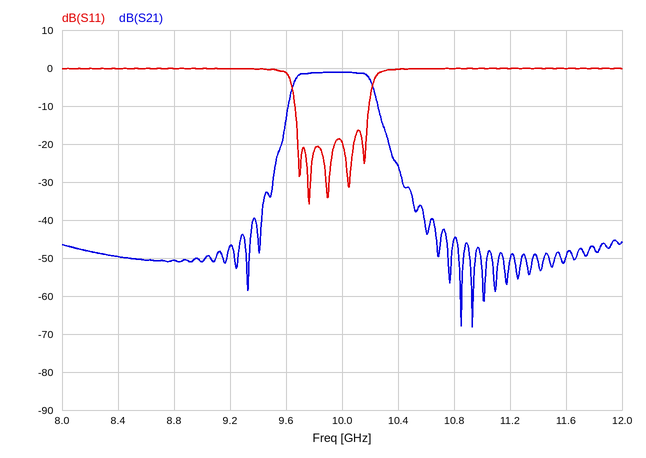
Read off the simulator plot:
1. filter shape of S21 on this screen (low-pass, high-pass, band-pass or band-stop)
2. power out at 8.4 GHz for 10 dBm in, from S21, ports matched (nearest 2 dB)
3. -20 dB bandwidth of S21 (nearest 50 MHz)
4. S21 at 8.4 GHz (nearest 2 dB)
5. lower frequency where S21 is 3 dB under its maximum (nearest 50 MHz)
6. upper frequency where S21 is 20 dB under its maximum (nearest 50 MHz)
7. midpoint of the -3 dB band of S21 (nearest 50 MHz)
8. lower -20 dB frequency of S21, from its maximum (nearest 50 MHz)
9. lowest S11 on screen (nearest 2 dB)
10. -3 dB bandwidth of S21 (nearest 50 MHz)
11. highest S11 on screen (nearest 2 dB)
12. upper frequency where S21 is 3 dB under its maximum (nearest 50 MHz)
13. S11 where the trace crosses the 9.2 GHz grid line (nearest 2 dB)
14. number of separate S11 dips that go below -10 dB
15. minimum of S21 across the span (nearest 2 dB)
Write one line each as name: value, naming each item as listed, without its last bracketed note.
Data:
filter shape of S21 on this screen: band-pass
power out at 8.4 GHz for 10 dBm in, from S21, ports matched: -40 dBm
-20 dB bandwidth of S21: 800 MHz
S21 at 8.4 GHz: -50 dB
lower frequency where S21 is 3 dB under its maximum: 9.65 GHz
upper frequency where S21 is 20 dB under its maximum: 10.35 GHz
midpoint of the -3 dB band of S21: 9.95 GHz
lower -20 dB frequency of S21, from its maximum: 9.55 GHz
lowest S11 on screen: -36 dB
-3 dB bandwidth of S21: 550 MHz
highest S11 on screen: 0 dB
upper frequency where S21 is 3 dB under its maximum: 10.20 GHz
S11 where the trace crosses the 9.2 GHz grid line: 0 dB
number of separate S11 dips that go below -10 dB: 5
minimum of S21 across the span: -68 dB
